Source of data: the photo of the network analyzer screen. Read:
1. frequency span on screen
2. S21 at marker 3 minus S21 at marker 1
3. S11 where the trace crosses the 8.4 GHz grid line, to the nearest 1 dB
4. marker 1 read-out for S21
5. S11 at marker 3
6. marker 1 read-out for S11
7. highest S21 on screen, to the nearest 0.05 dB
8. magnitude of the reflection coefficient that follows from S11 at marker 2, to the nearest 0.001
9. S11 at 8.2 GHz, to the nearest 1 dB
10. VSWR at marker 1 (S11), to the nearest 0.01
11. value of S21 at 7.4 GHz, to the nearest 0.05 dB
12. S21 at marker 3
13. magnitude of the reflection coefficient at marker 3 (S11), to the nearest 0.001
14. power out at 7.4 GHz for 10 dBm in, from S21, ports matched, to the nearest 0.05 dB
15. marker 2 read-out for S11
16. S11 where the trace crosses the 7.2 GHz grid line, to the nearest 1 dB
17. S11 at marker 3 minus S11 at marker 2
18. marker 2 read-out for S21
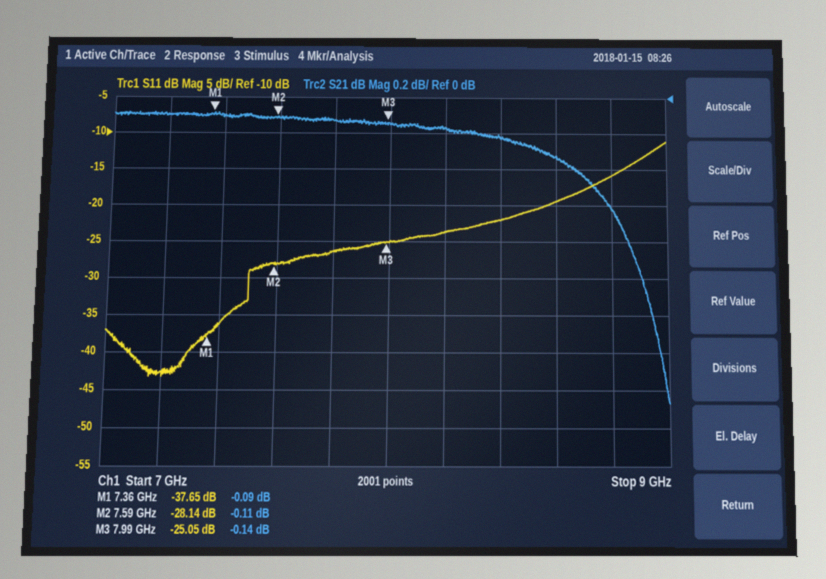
2 GHz
-0.05 dB
-22 dB
-0.09 dB
-25.05 dB
-37.65 dB
-0.10 dB
0.039
-24 dB
1.03
-0.10 dB
-0.14 dB
0.056
9.90 dBm
-28.14 dB
-43 dB
3.09 dB
-0.11 dB
